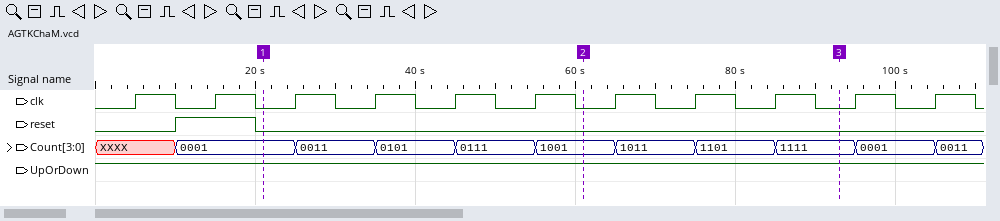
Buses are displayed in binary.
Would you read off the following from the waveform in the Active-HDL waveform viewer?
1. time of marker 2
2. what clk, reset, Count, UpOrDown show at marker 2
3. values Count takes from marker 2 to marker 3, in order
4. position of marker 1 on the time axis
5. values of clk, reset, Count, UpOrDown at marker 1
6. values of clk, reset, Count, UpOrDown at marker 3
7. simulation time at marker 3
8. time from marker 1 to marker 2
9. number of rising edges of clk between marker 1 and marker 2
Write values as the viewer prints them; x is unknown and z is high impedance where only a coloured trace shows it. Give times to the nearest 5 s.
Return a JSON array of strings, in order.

["60 s", "clk=0, reset=0, Count=1001, UpOrDown=1", "1001, 1011, 1101, 1111", "20 s", "clk=0, reset=0, Count=0001, UpOrDown=1", "clk=0, reset=0, Count=1111, UpOrDown=1", "95 s", "40 s", "4"]
